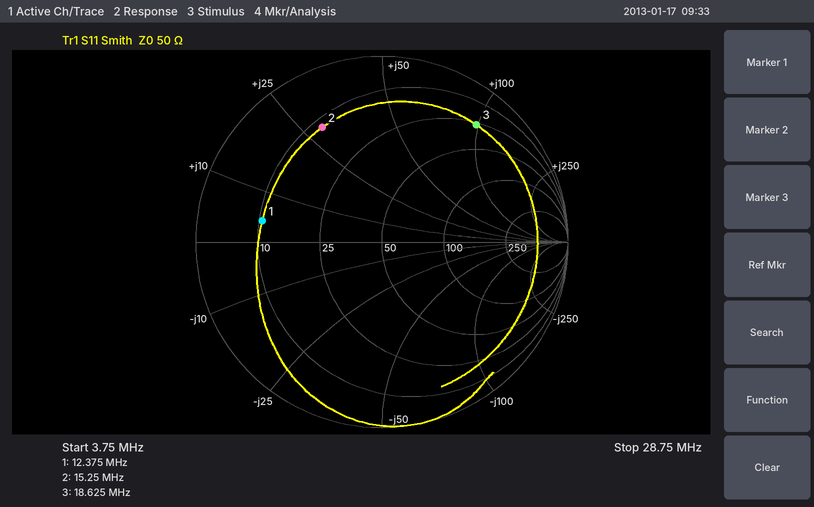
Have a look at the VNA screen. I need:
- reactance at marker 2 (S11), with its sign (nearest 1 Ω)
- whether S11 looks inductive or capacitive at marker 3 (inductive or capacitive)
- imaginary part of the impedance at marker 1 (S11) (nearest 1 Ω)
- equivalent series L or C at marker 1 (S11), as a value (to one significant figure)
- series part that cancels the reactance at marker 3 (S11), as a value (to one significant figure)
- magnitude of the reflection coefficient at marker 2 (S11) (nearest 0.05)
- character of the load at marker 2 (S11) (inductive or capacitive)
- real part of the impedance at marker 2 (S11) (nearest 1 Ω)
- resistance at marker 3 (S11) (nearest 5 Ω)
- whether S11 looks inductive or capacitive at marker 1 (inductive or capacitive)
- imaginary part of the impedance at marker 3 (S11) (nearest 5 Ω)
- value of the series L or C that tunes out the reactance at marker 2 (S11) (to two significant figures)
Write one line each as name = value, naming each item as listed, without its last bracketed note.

reactance at marker 2 (S11), with its sign = +29 Ω
whether S11 looks inductive or capacitive at marker 3 = inductive
imaginary part of the impedance at marker 1 (S11) = +4 Ω
equivalent series L or C at marker 1 (S11), as a value = 50 nH
series part that cancels the reactance at marker 3 (S11), as a value = 90 pF
magnitude of the reflection coefficient at marker 2 (S11) = 0.70
character of the load at marker 2 (S11) = inductive
real part of the impedance at marker 2 (S11) = 12 Ω
resistance at marker 3 (S11) = 25 Ω
whether S11 looks inductive or capacitive at marker 1 = inductive
imaginary part of the impedance at marker 3 (S11) = +100 Ω
value of the series L or C that tunes out the reactance at marker 2 (S11) = 360 pF
